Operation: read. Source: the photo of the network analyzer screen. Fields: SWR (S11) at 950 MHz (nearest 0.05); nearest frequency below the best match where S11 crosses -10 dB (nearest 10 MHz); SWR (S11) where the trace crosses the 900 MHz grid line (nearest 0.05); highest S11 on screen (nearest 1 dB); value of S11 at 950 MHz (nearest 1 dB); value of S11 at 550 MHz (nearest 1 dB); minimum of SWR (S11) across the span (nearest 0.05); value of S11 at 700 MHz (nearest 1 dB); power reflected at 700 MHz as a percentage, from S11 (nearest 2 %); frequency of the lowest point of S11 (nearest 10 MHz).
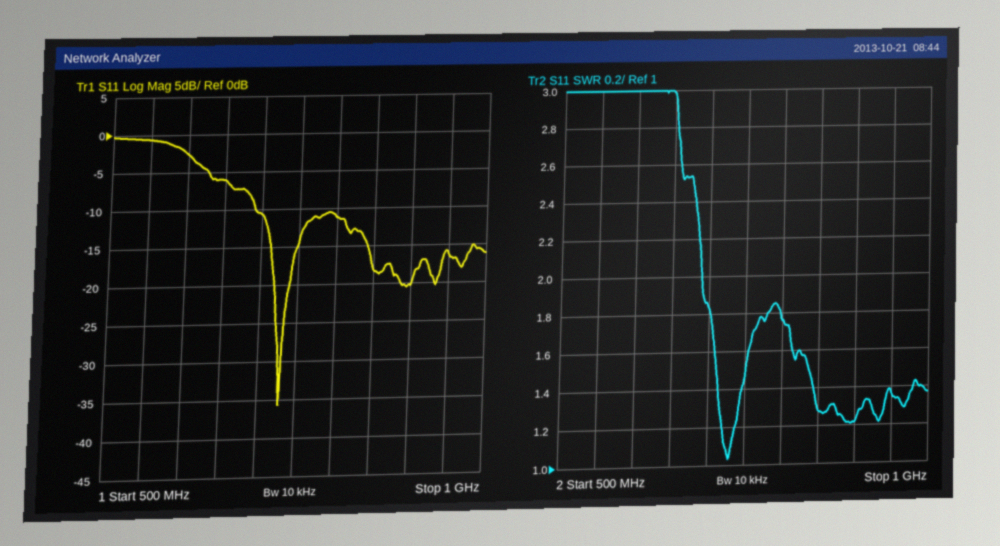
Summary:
1.35
690 MHz
1.20
0 dB
-16 dB
-1 dB
1.05
-11 dB
8 %
730 MHz
